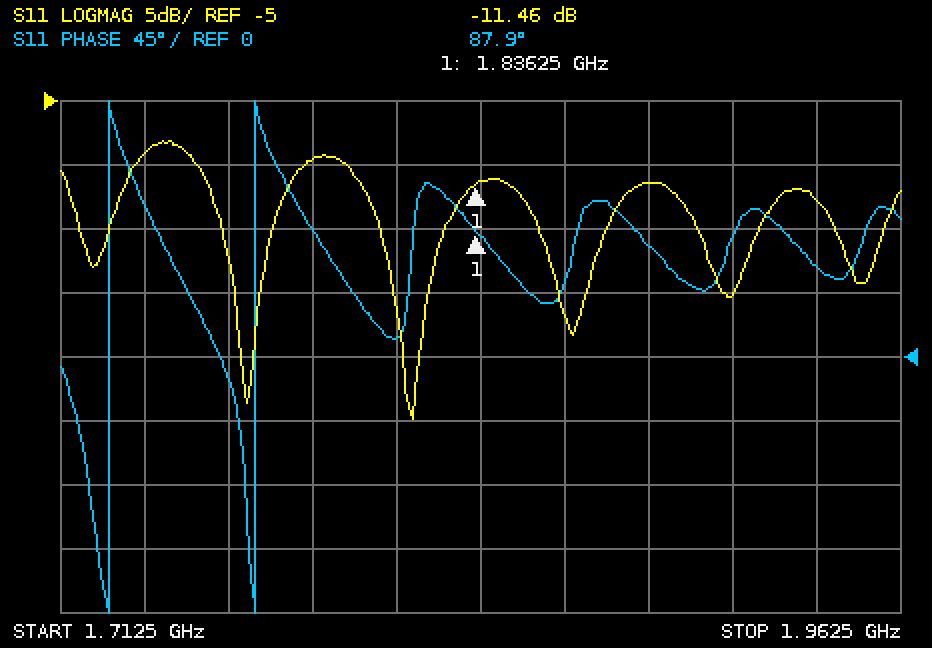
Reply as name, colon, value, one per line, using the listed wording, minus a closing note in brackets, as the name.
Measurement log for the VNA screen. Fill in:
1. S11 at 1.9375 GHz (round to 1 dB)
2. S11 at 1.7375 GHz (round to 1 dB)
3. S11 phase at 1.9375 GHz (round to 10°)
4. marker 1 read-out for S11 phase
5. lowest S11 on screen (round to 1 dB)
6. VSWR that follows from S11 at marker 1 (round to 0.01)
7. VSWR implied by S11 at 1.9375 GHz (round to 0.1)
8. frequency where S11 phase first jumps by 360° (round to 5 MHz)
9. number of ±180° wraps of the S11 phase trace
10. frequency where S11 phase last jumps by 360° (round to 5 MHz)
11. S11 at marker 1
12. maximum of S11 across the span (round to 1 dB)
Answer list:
S11 at 1.9375 GHz: -13 dB
S11 at 1.7375 GHz: -9 dB
S11 phase at 1.9375 GHz: 60°
marker 1 read-out for S11 phase: 87.9°
lowest S11 on screen: -30 dB
VSWR that follows from S11 at marker 1: 1.73
VSWR implied by S11 at 1.9375 GHz: 1.6
frequency where S11 phase first jumps by 360°: 1.725 GHz
number of ±180° wraps of the S11 phase trace: 2
frequency where S11 phase last jumps by 360°: 1.770 GHz
S11 at marker 1: -11.46 dB
maximum of S11 across the span: -8 dB
